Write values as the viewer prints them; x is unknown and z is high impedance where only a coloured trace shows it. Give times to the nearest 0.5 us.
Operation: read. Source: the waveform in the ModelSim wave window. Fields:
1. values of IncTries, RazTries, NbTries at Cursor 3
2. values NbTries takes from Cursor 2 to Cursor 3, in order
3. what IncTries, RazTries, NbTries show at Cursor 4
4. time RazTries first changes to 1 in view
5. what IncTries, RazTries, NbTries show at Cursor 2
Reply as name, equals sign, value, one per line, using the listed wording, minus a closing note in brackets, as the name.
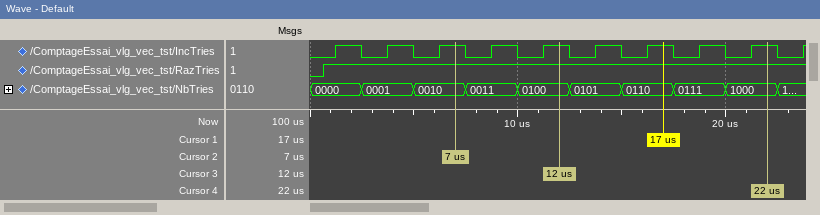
values of IncTries, RazTries, NbTries at Cursor 3 = IncTries=1, RazTries=1, NbTries=0100
values NbTries takes from Cursor 2 to Cursor 3, in order = 0010, 0011, 0100
what IncTries, RazTries, NbTries show at Cursor 4 = IncTries=1, RazTries=1, NbTries=1000
time RazTries first changes to 1 in view = 0.5 us
what IncTries, RazTries, NbTries show at Cursor 2 = IncTries=1, RazTries=1, NbTries=0010
